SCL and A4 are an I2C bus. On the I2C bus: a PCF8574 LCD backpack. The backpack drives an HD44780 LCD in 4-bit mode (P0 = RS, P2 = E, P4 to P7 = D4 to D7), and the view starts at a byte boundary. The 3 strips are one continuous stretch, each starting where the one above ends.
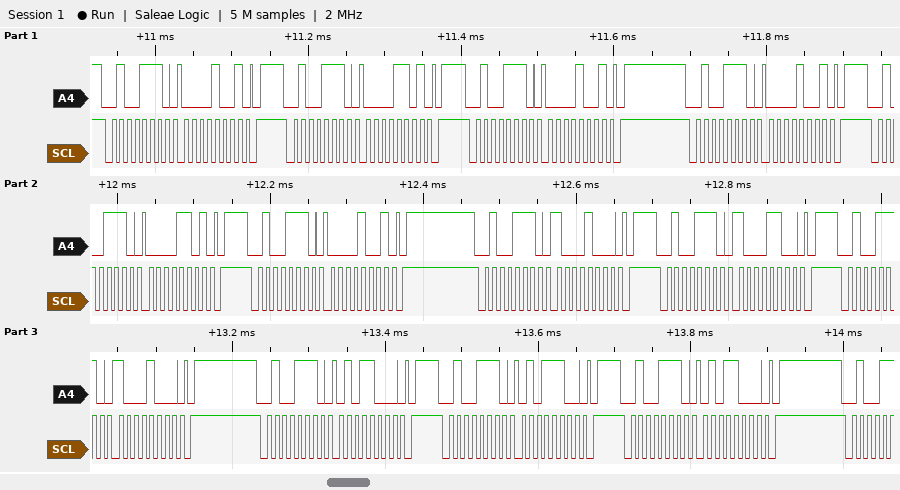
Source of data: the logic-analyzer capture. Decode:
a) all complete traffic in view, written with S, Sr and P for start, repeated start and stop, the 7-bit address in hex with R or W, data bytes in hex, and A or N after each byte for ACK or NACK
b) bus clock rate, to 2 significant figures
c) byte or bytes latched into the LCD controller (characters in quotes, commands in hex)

S 27W A 09 A P S 27W A 0D A P S 27W A 09 A P S 27W A 09 A P S 27W A 0D A P S 27W A 09 A P S 27W A 88 A P S 27W A 8C A P S 27W A 88 A P S 27W A 58 A P S 27W A 5C A P S 27W A 58 A P
100 kHz
data 0x00 0x85
